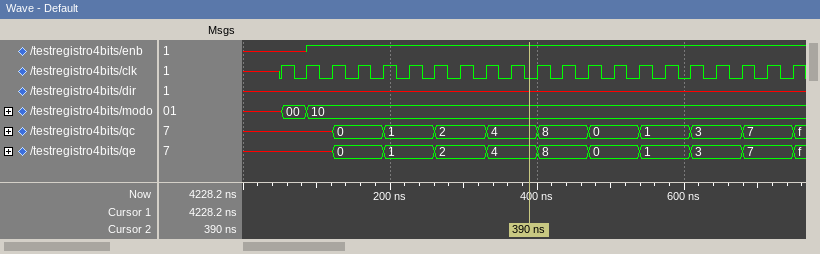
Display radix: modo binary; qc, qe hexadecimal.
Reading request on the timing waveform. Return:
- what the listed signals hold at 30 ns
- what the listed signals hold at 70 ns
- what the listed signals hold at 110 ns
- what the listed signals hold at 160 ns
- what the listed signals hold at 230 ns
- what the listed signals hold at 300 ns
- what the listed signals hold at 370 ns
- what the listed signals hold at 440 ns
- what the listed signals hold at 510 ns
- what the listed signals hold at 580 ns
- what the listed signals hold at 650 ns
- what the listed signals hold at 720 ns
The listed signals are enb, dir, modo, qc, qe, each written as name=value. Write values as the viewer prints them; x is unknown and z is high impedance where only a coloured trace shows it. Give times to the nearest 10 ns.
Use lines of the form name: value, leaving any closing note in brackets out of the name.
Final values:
what the listed signals hold at 30 ns: enb=x, dir=x, modo=x, qc=x, qe=x
what the listed signals hold at 70 ns: enb=x, dir=x, modo=00, qc=x, qe=x
what the listed signals hold at 110 ns: enb=1, dir=x, modo=10, qc=x, qe=x
what the listed signals hold at 160 ns: enb=1, dir=x, modo=10, qc=0, qe=0
what the listed signals hold at 230 ns: enb=1, dir=x, modo=10, qc=1, qe=1
what the listed signals hold at 300 ns: enb=1, dir=x, modo=10, qc=2, qe=2
what the listed signals hold at 370 ns: enb=1, dir=x, modo=10, qc=4, qe=4
what the listed signals hold at 440 ns: enb=1, dir=x, modo=10, qc=8, qe=8
what the listed signals hold at 510 ns: enb=1, dir=x, modo=10, qc=0, qe=0
what the listed signals hold at 580 ns: enb=1, dir=x, modo=10, qc=1, qe=1
what the listed signals hold at 650 ns: enb=1, dir=x, modo=10, qc=3, qe=3
what the listed signals hold at 720 ns: enb=1, dir=x, modo=10, qc=7, qe=7
